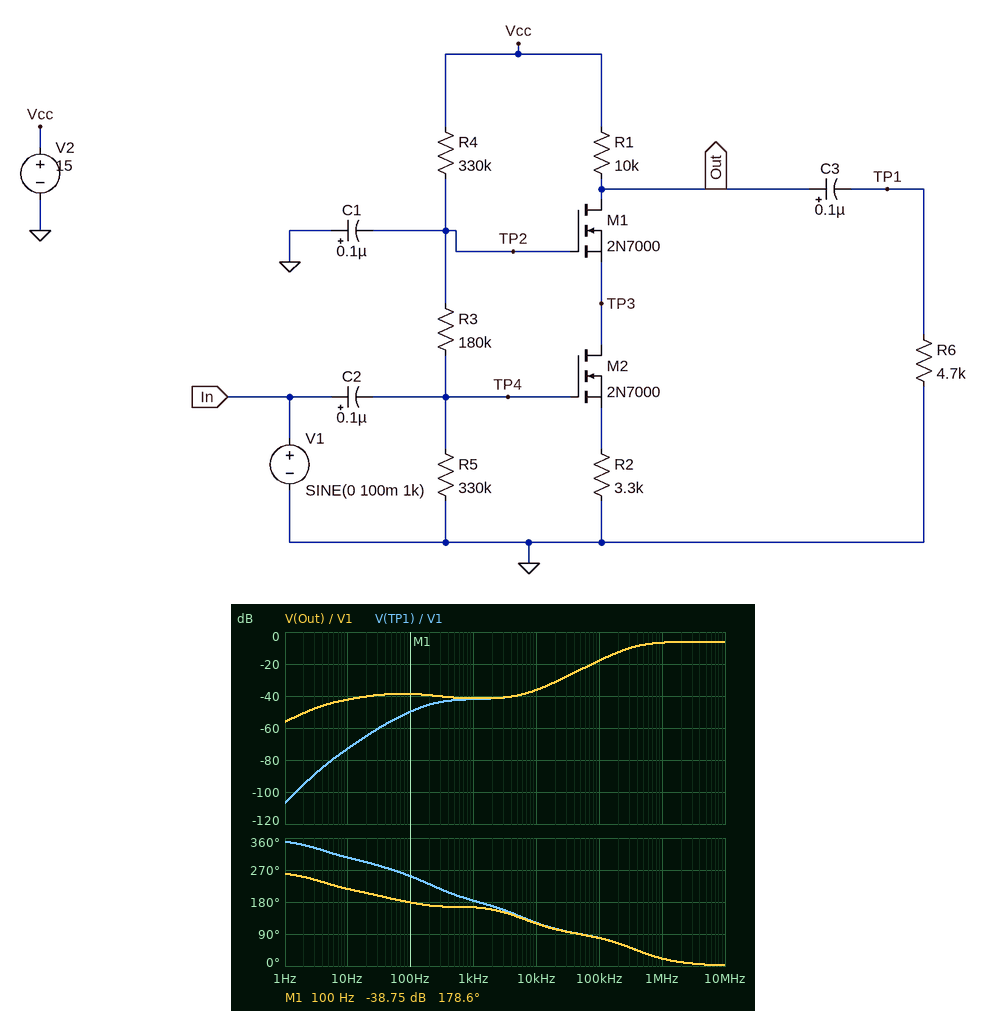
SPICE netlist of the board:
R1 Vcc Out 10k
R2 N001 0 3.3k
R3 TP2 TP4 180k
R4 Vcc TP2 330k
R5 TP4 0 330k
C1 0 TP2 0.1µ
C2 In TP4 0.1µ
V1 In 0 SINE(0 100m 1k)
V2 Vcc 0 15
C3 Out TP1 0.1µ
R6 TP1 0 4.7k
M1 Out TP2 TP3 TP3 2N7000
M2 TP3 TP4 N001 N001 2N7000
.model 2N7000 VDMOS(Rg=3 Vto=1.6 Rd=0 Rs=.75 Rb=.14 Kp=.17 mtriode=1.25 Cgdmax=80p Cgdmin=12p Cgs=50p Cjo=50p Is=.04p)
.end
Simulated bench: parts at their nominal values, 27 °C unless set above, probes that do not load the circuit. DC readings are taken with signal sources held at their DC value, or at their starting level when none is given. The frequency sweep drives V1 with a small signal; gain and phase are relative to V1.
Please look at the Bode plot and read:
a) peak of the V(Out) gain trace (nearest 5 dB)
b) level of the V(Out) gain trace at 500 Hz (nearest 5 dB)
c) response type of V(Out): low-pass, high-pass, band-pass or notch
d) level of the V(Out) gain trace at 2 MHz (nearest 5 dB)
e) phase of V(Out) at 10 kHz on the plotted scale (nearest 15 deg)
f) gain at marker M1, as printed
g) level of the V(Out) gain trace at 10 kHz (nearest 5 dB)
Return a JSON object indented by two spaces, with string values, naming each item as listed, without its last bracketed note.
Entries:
{
  "peak of the V(Out) gain trace": "-5 dB",
  "level of the V(Out) gain trace at 500 Hz": "-40 dB",
  "response type of V(Out): low-pass, high-pass, band-pass or notch": "high-pass",
  "level of the V(Out) gain trace at 2 MHz": "-5 dB",
  "phase of V(Out) at 10 kHz on the plotted scale": "120 deg",
  "gain at marker M1, as printed": "-38.75 dB",
  "level of the V(Out) gain trace at 10 kHz": "-35 dB"
}
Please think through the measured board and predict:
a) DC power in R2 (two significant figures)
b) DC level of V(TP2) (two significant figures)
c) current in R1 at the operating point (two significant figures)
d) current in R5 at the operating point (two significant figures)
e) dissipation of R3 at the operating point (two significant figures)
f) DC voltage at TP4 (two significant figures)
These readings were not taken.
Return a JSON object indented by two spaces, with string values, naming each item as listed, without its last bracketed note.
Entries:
{
  "DC power in R2": "4.2 mW",
  "DC level of V(TP2)": "9.1 V",
  "current in R1 at the operating point": "1.1 mA",
  "current in R5 at the operating point": "18 µA",
  "dissipation of R3 at the operating point": "57 µW",
  "DC voltage at TP4": "5.9 V"
}
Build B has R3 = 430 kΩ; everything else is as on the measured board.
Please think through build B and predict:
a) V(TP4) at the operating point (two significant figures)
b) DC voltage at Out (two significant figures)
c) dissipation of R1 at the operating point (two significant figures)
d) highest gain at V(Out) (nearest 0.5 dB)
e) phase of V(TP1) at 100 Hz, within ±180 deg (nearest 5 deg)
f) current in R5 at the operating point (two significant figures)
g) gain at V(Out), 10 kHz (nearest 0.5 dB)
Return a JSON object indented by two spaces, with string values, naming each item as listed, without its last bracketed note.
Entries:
{
  "V(TP4) at the operating point": "4.5 V",
  "DC voltage at Out": "6.3 V",
  "dissipation of R1 at the operating point": "7.6 mW",
  "highest gain at V(Out)": "8.5 dB",
  "phase of V(TP1) at 100 Hz, within ±180 deg": "-130 deg",
  "current in R5 at the operating point": "14 µA",
  "gain at V(Out), 10 kHz": "-0.5 dB"
}
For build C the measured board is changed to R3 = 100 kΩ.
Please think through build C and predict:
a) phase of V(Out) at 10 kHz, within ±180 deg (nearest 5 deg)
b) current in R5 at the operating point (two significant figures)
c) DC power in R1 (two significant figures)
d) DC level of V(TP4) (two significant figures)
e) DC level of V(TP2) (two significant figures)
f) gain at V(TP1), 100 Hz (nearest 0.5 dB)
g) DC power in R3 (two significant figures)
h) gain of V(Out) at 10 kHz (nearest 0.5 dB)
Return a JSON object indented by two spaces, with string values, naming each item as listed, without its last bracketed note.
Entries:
{
  "phase of V(Out) at 10 kHz, within ±180 deg": "95 deg",
  "current in R5 at the operating point": "20 µA",
  "DC power in R1": "13 mW",
  "DC level of V(TP4)": "6.5 V",
  "DC level of V(TP2)": "8.5 V",
  "gain at V(TP1), 100 Hz": "-63.0 dB",
  "DC power in R3": "39 µW",
  "gain of V(Out) at 10 kHz": "-37.5 dB"
}
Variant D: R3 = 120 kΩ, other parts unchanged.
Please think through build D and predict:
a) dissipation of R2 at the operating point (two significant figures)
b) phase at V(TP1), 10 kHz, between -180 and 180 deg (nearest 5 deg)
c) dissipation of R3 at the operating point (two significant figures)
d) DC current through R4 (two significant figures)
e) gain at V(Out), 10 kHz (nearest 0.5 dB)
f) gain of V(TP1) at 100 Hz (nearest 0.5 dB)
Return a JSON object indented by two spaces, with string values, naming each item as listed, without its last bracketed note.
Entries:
{
  "dissipation of R2 at the operating point": "4.2 mW",
  "phase at V(TP1), 10 kHz, between -180 and 180 deg": "100 deg",
  "dissipation of R3 at the operating point": "44 µW",
  "DC current through R4": "19 µA",
  "gain at V(Out), 10 kHz": "-37.5 dB",
  "gain of V(TP1) at 100 Hz": "-60.0 dB"
}
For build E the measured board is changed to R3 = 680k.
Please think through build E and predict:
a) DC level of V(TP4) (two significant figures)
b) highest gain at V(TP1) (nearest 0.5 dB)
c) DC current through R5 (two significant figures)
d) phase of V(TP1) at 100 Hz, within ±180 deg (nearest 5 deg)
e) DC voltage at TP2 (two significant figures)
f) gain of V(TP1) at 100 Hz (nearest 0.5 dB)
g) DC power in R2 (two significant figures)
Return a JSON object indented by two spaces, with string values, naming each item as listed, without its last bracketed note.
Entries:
{
  "DC level of V(TP4)": "3.7 V",
  "highest gain at V(TP1)": "-0.5 dB",
  "DC current through R5": "11 µA",
  "phase of V(TP1) at 100 Hz, within ±180 deg": "-130 deg",
  "DC voltage at TP2": "11 V",
  "gain of V(TP1) at 100 Hz": "-4.0 dB",
  "DC power in R2": "1.3 mW"
}
